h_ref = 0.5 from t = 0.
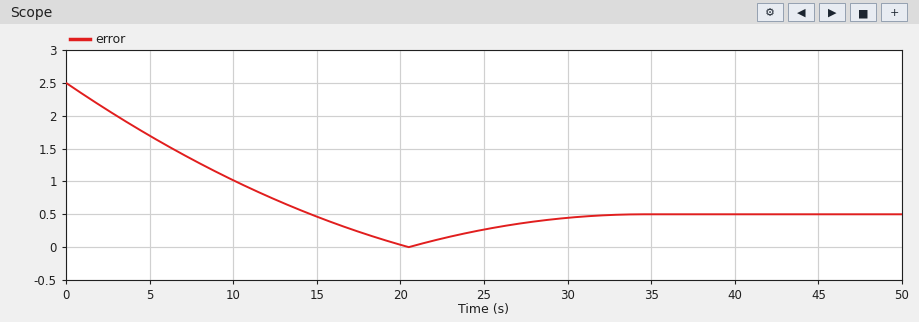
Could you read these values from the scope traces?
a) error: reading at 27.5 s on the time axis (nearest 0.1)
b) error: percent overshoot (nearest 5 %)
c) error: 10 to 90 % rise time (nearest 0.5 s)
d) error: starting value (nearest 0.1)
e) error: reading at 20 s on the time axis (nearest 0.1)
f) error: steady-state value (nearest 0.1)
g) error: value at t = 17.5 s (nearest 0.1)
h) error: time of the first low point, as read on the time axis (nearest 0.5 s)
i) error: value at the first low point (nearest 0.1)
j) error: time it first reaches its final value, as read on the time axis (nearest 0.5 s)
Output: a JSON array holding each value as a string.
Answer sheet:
["0.4", "25 %", "11.5 s", "2.5", "0.0", "0.5", "0.2", "20.5 s", "0.0", "14.5 s"]
